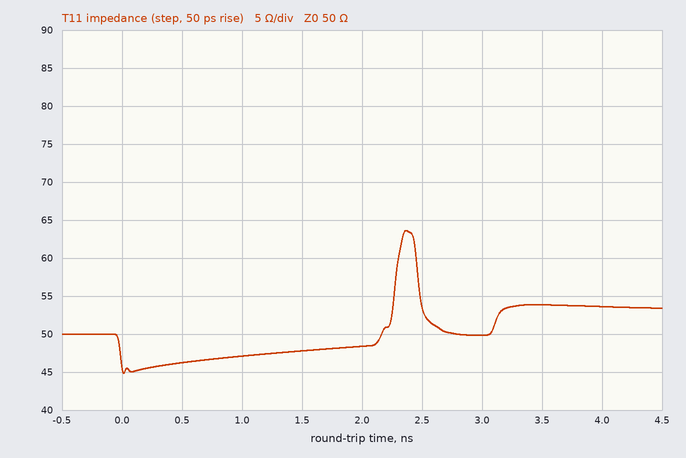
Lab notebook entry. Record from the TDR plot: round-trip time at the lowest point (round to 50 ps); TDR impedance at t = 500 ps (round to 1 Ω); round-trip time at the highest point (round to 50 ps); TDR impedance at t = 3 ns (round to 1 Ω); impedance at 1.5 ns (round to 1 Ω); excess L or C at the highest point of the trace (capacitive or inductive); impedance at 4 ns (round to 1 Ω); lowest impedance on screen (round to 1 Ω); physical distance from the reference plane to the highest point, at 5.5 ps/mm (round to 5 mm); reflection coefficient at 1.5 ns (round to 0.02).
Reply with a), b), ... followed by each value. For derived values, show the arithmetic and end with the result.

a) 0 ps
b) 46 Ω
c) 2.35 ns
d) 50 Ω
e) 48 Ω
f) inductive
g) 54 Ω
h) 45 Ω
i) 2.35 ns / 2 / 5.5 ps/mm ≈ 214 mm, so 215 mm to the nearest 5 mm
j) (48 − 50)/(48 + 50) ≈ -0.02
